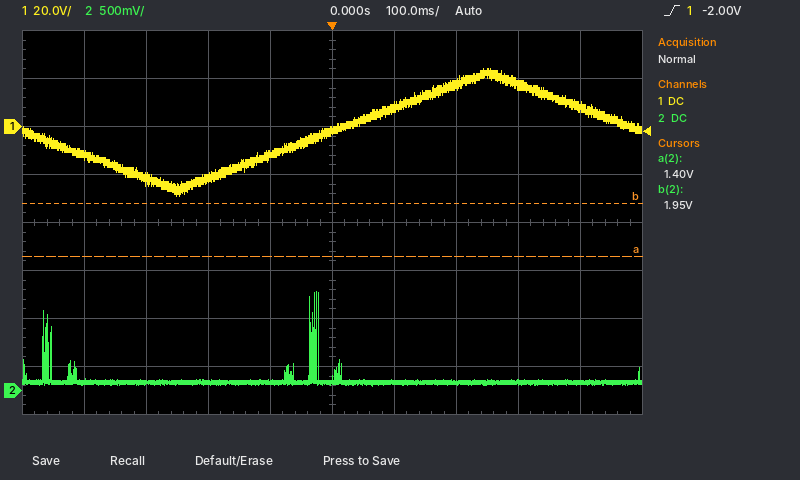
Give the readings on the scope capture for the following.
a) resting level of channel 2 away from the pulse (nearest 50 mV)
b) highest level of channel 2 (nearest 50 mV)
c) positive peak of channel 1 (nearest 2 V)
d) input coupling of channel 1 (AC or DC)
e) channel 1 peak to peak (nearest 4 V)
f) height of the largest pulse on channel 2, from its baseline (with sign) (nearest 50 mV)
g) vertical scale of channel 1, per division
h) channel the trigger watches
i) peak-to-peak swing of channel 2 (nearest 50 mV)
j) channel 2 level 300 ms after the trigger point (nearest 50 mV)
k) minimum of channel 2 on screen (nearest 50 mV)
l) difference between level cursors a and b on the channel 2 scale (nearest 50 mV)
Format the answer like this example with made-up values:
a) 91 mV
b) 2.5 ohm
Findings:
a) 100 mV
b) 1.05 V
c) 24 V
d) DC
e) 52 V
f) +950 mV
g) 20 V
h) channel 1
i) 1.00 V
j) 100 mV
k) 50 mV
l) 550 mV
